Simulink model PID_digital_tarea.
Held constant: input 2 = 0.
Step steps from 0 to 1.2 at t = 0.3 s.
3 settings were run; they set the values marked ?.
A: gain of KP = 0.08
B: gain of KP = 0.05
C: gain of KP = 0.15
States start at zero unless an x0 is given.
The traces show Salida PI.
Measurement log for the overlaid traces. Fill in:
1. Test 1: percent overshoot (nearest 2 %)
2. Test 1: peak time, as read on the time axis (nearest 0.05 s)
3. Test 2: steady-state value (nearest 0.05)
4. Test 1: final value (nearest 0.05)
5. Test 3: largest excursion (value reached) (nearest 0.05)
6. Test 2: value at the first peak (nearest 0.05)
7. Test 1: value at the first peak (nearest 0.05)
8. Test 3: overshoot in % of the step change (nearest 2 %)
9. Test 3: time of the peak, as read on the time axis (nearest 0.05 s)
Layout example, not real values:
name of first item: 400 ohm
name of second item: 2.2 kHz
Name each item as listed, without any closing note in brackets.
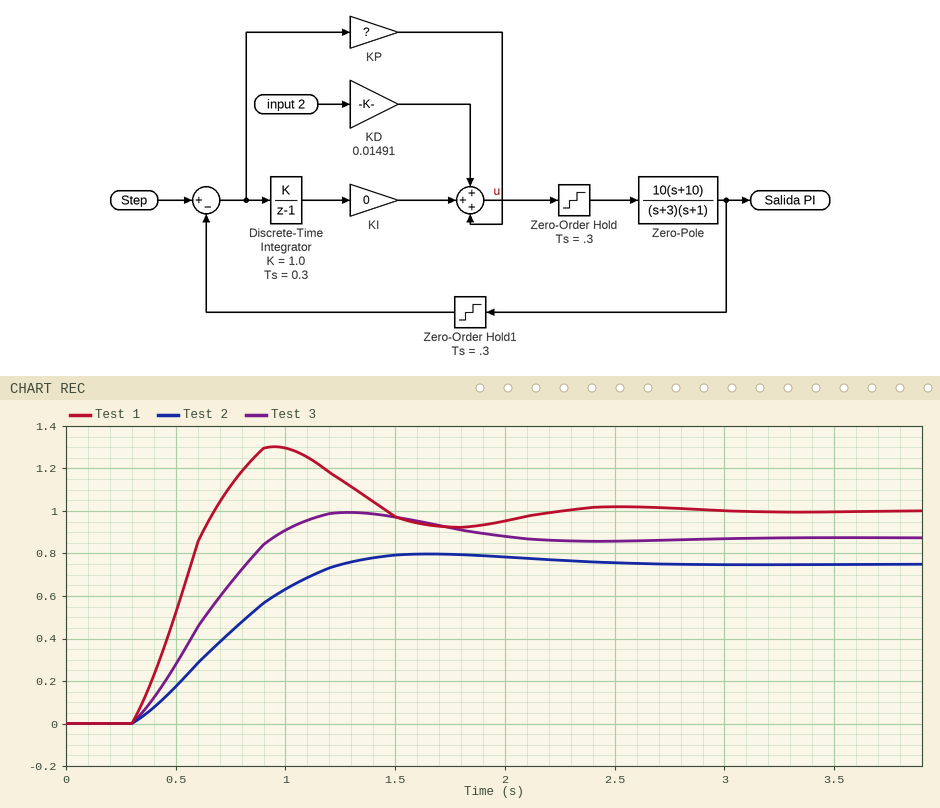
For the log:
Test 1: percent overshoot: 30 %
Test 1: peak time, as read on the time axis: 0.95 s
Test 2: steady-state value: 0.75
Test 1: final value: 1.00
Test 3: largest excursion (value reached): 1.00
Test 2: value at the first peak: 0.80
Test 1: value at the first peak: 1.30
Test 3: overshoot in % of the step change: 14 %
Test 3: time of the peak, as read on the time axis: 1.30 s
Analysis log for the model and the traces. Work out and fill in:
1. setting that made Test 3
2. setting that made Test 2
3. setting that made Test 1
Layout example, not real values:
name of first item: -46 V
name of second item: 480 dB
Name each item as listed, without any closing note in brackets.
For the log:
setting that made Test 3: A
setting that made Test 2: B
setting that made Test 1: C
